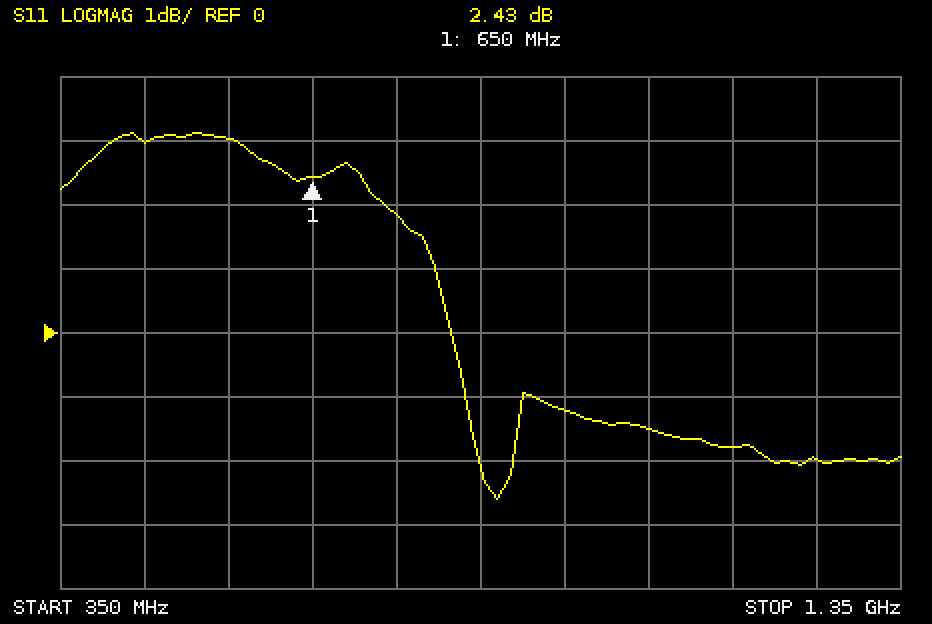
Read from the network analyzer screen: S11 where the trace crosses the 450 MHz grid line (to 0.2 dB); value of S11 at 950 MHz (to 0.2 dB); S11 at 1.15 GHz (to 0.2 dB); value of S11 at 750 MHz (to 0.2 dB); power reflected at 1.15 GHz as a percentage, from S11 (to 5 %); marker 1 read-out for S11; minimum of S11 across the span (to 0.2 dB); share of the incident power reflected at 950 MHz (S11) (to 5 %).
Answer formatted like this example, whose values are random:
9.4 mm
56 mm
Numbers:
3.0 dB
-1.2 dB
-1.8 dB
1.8 dB
65 %
2.43 dB
-2.6 dB
75 %
